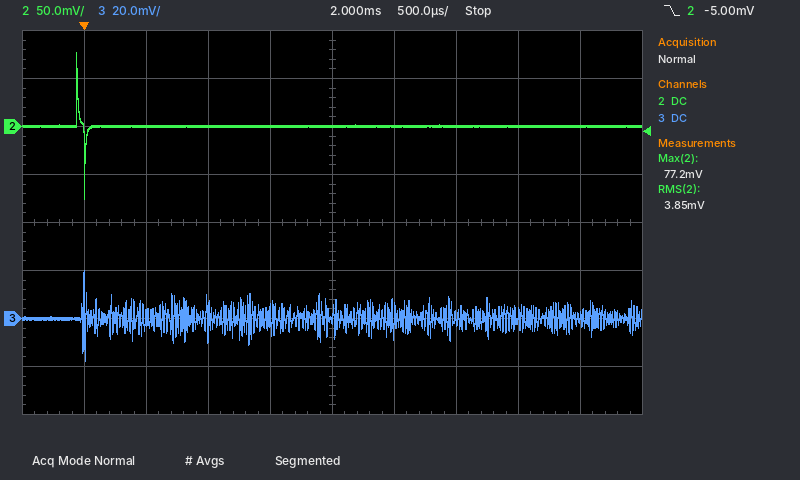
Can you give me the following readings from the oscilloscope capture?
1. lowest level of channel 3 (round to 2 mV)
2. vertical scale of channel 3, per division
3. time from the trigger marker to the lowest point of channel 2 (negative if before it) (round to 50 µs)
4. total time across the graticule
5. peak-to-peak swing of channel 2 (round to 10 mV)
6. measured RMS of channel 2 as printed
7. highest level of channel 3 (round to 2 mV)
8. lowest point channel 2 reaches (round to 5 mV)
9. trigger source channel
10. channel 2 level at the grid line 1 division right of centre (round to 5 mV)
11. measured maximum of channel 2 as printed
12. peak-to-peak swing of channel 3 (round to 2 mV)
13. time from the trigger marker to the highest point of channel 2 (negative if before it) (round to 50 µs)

-18 mV
20 mV
0 µs
5 ms
150 mV
3.85 mV
20 mV
-75 mV
channel 2
0 mV
77.2 mV
38 mV
-50 µs
